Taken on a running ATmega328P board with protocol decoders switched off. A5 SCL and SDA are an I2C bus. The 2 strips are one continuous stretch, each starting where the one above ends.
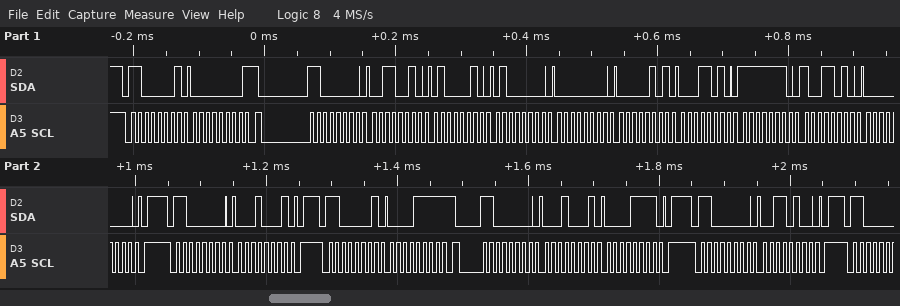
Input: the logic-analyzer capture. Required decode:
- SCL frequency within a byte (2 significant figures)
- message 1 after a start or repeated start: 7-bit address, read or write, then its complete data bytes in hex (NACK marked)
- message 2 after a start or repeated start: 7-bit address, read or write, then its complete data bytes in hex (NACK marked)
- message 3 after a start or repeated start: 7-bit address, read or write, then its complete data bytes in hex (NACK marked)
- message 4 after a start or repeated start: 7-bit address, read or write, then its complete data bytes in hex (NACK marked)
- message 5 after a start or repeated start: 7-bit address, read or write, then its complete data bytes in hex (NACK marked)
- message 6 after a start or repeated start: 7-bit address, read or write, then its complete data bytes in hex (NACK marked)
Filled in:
100 kHz
0x60 read: 00 NACK
0x60 write: 32 42 40 00 05 1A FE 9A 00
0x60 write: 11
0x60 read: 0F NACK
0x60 write: 11 0F
0x60 write: 34
